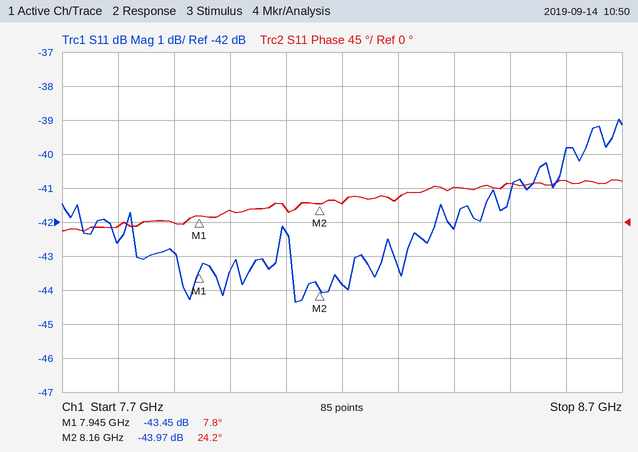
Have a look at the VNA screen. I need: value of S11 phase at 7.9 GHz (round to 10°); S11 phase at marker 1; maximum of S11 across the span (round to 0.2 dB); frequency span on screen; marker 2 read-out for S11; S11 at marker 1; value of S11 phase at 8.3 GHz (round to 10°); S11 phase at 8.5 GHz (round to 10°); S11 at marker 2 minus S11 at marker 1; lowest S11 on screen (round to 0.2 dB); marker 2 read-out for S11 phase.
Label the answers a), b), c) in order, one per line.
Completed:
a) 0°
b) 7.8°
c) -39.0 dB
d) 1 GHz
e) -43.97 dB
f) -43.45 dB
g) 30°
h) 50°
i) -0.52 dB
j) -44.4 dB
k) 24.2°
